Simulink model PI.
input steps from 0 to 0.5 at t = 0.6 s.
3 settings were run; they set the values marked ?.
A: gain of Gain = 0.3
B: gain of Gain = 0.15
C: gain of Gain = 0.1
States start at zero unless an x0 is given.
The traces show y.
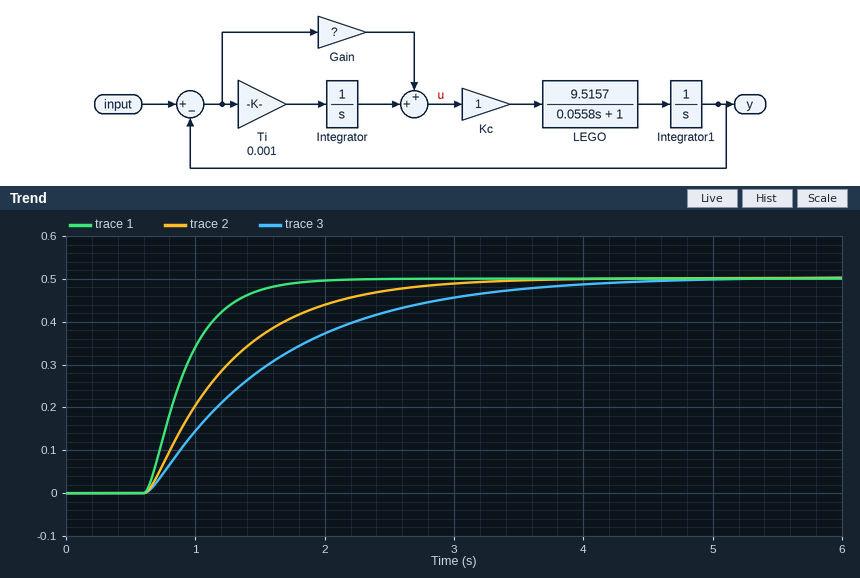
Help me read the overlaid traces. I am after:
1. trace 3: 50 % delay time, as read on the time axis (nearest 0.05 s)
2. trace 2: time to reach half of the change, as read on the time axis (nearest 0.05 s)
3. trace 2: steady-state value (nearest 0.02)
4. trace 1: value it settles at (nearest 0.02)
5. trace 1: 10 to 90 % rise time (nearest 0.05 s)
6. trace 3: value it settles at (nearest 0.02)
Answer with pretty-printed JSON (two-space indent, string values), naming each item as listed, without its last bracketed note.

{
  "trace 3: 50 % delay time, as read on the time axis": "1.35 s",
  "trace 2: time to reach half of the change, as read on the time axis": "1.10 s",
  "trace 2: steady-state value": "0.50",
  "trace 1: value it settles at": "0.50",
  "trace 1: 10 to 90 % rise time": "0.65 s",
  "trace 3: value it settles at": "0.50"
}
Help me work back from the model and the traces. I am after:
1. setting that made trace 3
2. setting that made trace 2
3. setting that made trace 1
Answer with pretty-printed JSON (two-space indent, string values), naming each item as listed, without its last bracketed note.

{
  "setting that made trace 3": "C",
  "setting that made trace 2": "B",
  "setting that made trace 1": "A"
}
